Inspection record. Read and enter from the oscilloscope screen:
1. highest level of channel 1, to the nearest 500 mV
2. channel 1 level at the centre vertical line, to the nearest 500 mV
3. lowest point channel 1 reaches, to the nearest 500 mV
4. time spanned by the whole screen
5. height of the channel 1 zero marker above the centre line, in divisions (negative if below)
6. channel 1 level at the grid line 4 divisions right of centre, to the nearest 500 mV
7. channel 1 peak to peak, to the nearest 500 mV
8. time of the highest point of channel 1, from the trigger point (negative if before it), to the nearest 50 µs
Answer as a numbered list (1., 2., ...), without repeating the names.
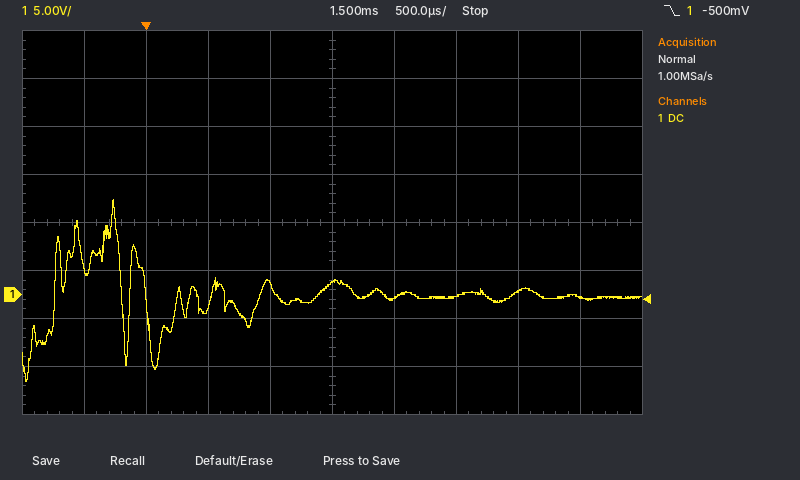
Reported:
1. 10.0 V
2. 1.5 V
3. -9.0 V
4. 5 ms
5. -1.5 div
6. -500 mV
7. 19.0 V
8. -250 µs
